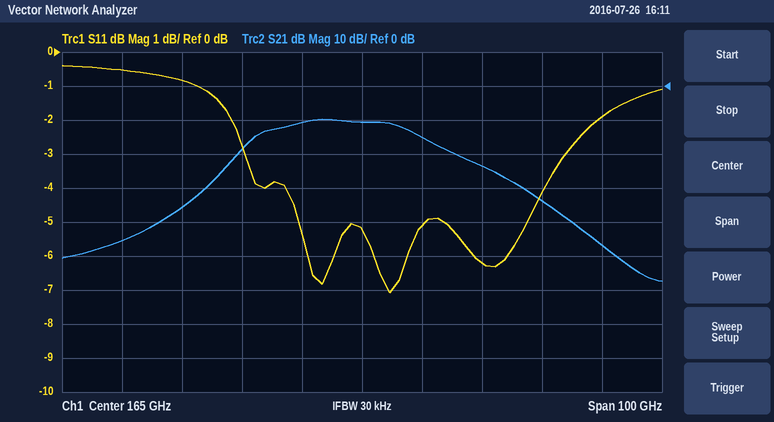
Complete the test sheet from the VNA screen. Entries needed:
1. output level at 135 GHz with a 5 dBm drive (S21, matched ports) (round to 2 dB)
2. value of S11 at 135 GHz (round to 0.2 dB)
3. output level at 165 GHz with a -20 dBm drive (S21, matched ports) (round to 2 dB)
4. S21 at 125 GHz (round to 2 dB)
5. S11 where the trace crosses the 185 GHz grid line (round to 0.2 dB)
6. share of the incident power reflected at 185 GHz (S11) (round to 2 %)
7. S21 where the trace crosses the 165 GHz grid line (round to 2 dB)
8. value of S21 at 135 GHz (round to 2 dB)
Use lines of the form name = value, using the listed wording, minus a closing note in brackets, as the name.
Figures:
output level at 135 GHz with a 5 dBm drive (S21, matched ports) = -30 dBm
value of S11 at 135 GHz = -0.8 dB
output level at 165 GHz with a -20 dBm drive (S21, matched ports) = -30 dBm
S21 at 125 GHz = -46 dB
S11 where the trace crosses the 185 GHz grid line = -6.2 dB
share of the incident power reflected at 185 GHz (S11) = 24 %
S21 where the trace crosses the 165 GHz grid line = -10 dB
value of S21 at 135 GHz = -36 dB
